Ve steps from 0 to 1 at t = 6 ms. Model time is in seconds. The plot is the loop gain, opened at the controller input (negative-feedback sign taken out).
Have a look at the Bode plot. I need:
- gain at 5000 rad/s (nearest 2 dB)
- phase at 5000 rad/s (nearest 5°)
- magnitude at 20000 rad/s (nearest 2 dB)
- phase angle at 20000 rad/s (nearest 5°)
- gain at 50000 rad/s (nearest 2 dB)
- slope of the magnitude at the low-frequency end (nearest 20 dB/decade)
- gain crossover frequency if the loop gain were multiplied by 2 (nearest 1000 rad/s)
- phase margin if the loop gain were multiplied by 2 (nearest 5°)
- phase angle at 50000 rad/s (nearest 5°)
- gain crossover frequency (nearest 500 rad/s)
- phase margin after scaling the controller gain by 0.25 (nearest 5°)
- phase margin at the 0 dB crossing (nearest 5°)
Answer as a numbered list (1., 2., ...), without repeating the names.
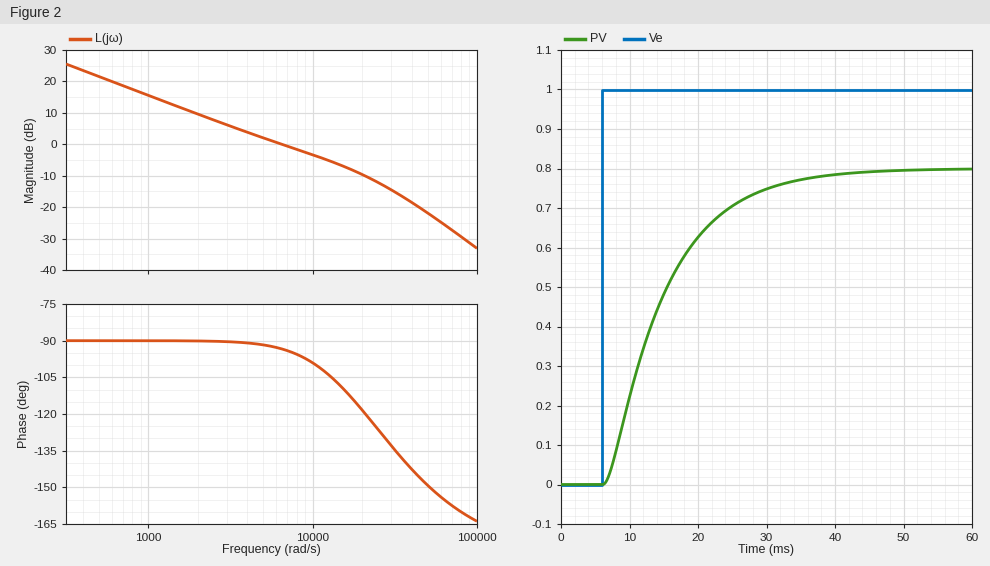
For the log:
1. 2 dB
2. -90°
3. -10 dB
4. -120°
5. -22 dB
6. -20 dB/decade
7. 14000 rad/s
8. 75°
9. -150°
10. 6500 rad/s
11. 90°
12. 85°
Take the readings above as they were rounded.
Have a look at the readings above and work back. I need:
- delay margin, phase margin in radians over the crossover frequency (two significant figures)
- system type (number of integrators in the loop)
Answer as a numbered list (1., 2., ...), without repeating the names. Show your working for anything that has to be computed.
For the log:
1. 85 × π / 180 / 6500 = 0.00023 s
2. 1
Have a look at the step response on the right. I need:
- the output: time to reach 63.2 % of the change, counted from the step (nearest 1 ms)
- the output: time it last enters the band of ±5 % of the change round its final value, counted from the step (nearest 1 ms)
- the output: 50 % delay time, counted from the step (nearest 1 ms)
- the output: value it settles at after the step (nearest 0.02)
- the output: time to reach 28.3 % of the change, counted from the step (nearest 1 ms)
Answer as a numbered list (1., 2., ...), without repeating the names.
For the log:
1. 10 ms
2. 26 ms
3. 7 ms
4. 0.80
5. 4 ms
